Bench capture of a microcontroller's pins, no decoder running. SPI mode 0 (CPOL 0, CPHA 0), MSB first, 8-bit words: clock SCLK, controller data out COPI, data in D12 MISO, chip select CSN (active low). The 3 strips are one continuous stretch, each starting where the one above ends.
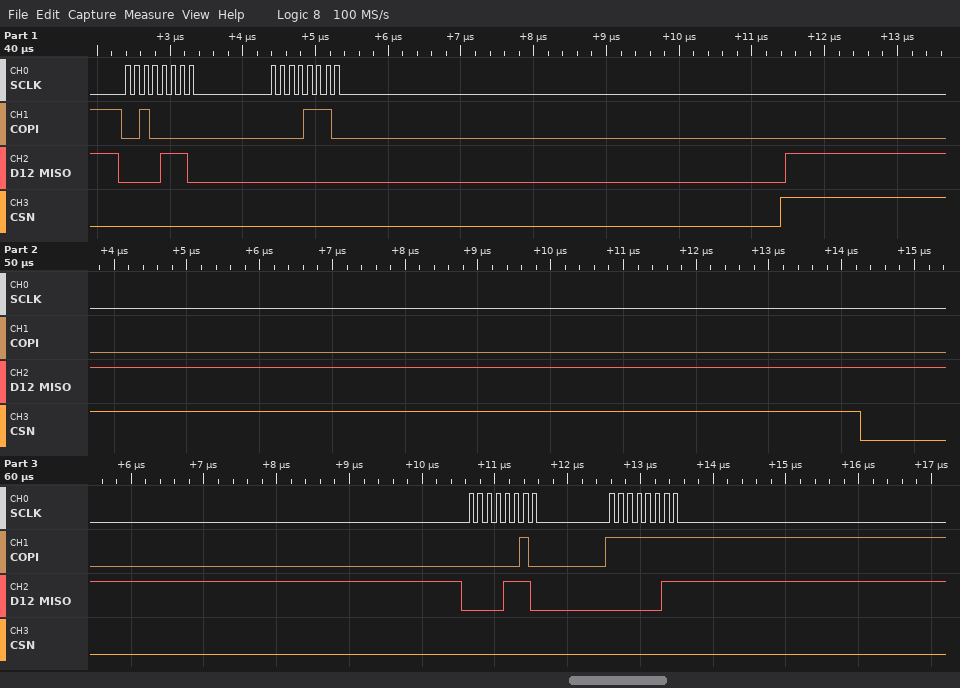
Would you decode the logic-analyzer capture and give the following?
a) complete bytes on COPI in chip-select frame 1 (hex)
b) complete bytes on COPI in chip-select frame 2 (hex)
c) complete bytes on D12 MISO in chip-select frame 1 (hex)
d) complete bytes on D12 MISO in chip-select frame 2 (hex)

0x20 0x0E
0x02 0xFF
0x0E 0x00
0x0E 0x03
